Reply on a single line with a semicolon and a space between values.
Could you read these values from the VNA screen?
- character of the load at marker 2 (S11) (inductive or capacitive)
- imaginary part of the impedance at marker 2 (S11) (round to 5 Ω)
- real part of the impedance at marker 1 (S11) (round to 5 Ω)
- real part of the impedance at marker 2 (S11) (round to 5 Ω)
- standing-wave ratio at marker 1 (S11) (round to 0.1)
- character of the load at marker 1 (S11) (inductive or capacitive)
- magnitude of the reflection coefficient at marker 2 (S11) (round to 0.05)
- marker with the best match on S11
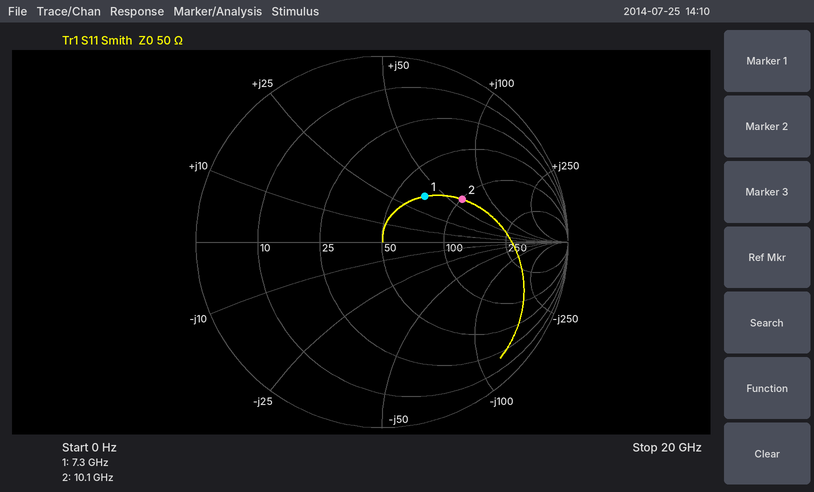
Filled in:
inductive; +60 Ω; 70 Ω; 100 Ω; 2.0; inductive; 0.50; marker 1
